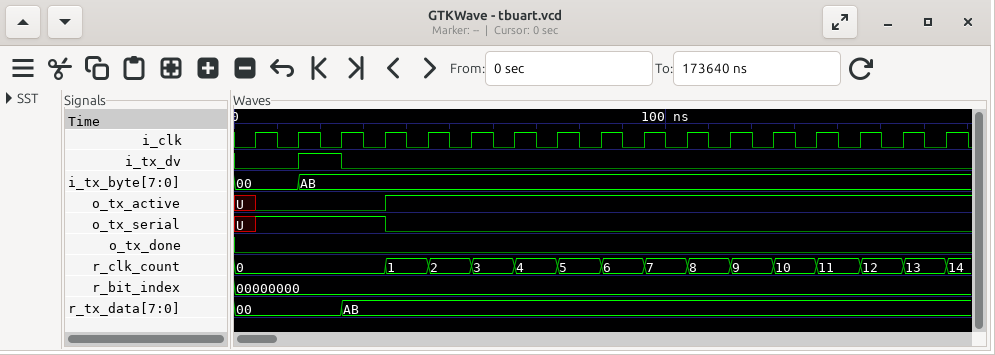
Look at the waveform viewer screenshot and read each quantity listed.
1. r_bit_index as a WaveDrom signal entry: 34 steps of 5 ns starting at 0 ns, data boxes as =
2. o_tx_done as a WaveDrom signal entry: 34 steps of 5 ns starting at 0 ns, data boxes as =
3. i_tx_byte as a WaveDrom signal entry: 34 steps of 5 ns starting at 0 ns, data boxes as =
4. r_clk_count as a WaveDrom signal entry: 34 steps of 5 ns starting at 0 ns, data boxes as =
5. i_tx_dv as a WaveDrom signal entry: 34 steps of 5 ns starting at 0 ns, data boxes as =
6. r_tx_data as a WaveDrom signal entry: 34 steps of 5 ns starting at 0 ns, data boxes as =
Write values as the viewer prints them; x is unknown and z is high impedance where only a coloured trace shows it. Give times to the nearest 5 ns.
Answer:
{name: 'r_bit_index', wave: '=.................................', data: '00000000'}
{name: 'o_tx_done', wave: '0.................................'}
{name: 'i_tx_byte', wave: '=..=..............................', data: '00 AB'}
{name: 'r_clk_count', wave: '=......=.=.=.=.=.=.=.=.=.=.=.=.=.=', data: '0 1 2 3 4 5 6 7 8 9 10 11 12 13 14'}
{name: 'i_tx_dv', wave: '0..1.0............................'}
{name: 'r_tx_data', wave: '=....=............................', data: '00 AB'}
